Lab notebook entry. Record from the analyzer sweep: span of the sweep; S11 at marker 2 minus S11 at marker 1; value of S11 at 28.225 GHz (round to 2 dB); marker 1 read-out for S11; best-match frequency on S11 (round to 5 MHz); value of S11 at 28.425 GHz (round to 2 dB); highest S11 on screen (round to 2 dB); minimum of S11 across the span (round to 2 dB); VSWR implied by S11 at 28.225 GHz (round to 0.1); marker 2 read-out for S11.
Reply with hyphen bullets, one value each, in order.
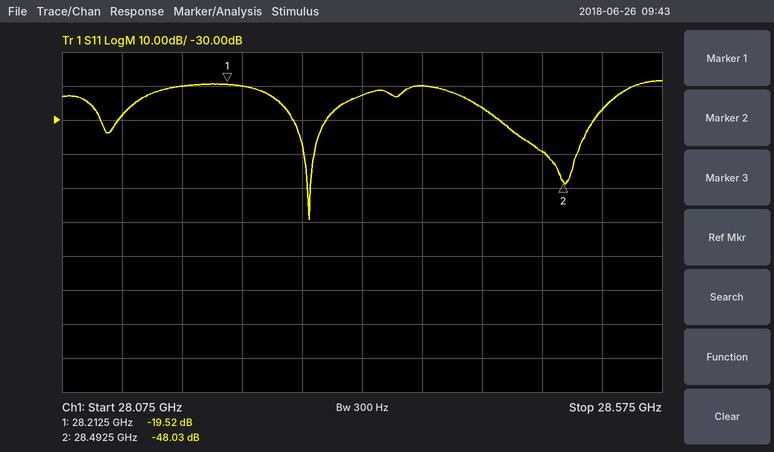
- 500 MHz
- -28.51 dB
- -20 dB
- -19.52 dB
- 28.280 GHz
- -26 dB
- -18 dB
- -60 dB
- 1.2
- -48.03 dB
